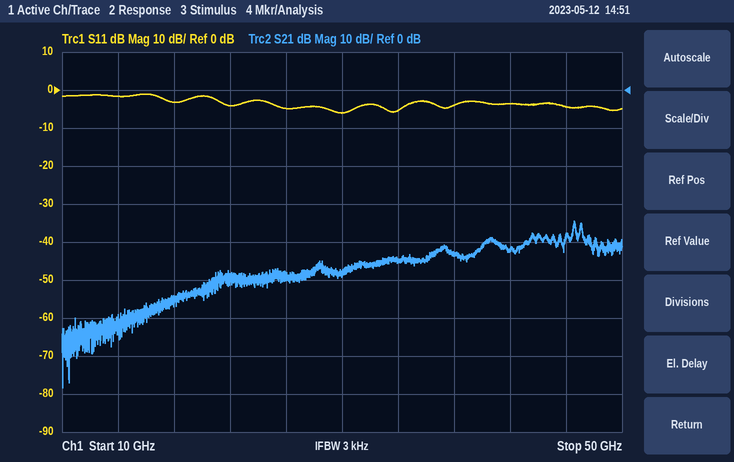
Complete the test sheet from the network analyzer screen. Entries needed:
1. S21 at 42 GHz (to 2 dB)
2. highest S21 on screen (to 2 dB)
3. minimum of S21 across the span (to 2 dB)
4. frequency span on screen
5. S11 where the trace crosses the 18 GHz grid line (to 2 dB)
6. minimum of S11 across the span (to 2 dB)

-42 dB
-34 dB
-78 dB
40 GHz
-4 dB
-6 dB
